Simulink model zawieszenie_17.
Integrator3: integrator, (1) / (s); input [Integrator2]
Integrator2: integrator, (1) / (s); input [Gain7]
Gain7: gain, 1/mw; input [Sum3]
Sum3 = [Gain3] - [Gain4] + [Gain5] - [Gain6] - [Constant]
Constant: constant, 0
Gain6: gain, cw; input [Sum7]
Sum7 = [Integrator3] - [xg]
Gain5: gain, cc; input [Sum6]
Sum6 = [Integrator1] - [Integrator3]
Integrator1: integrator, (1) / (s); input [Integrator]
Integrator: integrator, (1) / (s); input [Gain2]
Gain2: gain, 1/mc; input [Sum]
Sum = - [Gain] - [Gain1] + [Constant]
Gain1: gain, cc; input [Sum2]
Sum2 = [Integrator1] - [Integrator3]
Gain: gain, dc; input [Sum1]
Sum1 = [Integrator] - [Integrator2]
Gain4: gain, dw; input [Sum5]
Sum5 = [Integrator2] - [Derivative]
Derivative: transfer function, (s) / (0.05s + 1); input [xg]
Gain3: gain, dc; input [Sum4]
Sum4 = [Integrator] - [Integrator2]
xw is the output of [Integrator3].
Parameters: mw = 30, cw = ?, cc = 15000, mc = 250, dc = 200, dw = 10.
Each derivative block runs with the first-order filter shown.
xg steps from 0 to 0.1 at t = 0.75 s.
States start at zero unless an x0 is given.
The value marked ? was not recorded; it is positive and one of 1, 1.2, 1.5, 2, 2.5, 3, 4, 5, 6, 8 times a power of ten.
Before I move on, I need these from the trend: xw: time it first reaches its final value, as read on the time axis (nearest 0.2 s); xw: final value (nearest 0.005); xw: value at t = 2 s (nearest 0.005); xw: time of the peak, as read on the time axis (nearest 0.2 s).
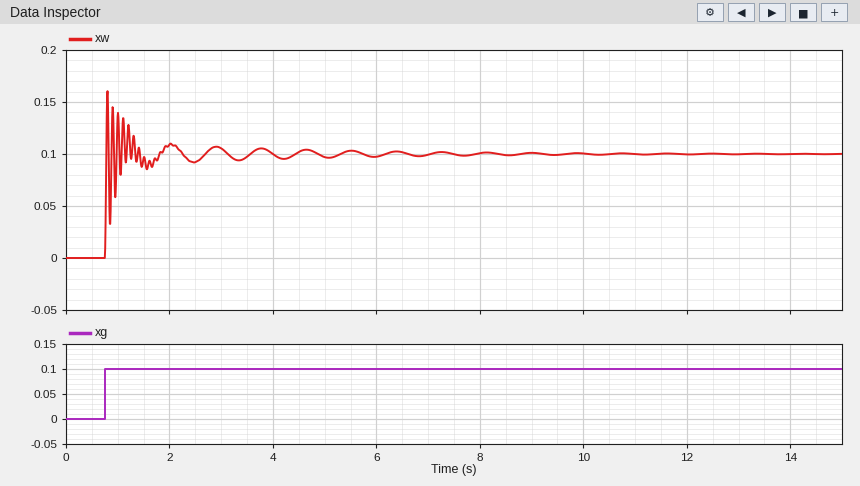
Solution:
0.8 s
0.100
0.110
0.8 s
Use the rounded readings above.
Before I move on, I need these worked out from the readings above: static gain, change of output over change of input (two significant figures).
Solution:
1.0
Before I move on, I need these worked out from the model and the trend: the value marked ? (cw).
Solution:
100000
